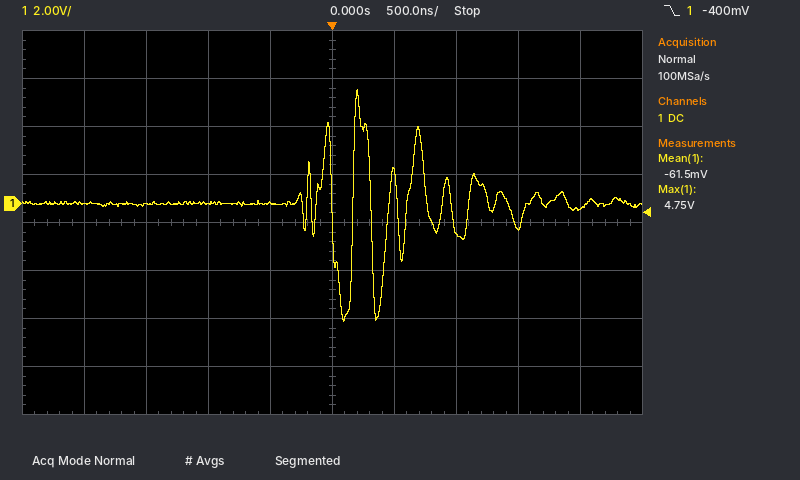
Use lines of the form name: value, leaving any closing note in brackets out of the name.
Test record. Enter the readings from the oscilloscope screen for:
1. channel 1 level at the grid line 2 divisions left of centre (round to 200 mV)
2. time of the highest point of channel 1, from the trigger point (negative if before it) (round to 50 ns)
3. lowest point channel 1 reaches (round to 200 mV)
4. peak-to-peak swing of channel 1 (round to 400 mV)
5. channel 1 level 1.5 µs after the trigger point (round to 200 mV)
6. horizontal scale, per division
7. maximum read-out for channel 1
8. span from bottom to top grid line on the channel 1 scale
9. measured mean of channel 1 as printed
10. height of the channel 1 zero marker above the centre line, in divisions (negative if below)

channel 1 level at the grid line 2 divisions left of centre: 0.0 V
time of the highest point of channel 1, from the trigger point (negative if before it): +200 ns
lowest point channel 1 reaches: -5.0 V
peak-to-peak swing of channel 1: 9.6 V
channel 1 level 1.5 µs after the trigger point: -1.0 V
horizontal scale, per division: 500 ns
maximum read-out for channel 1: 4.75 V
span from bottom to top grid line on the channel 1 scale: 16 V
measured mean of channel 1 as printed: -61.5 mV
height of the channel 1 zero marker above the centre line, in divisions: +0.4 div
